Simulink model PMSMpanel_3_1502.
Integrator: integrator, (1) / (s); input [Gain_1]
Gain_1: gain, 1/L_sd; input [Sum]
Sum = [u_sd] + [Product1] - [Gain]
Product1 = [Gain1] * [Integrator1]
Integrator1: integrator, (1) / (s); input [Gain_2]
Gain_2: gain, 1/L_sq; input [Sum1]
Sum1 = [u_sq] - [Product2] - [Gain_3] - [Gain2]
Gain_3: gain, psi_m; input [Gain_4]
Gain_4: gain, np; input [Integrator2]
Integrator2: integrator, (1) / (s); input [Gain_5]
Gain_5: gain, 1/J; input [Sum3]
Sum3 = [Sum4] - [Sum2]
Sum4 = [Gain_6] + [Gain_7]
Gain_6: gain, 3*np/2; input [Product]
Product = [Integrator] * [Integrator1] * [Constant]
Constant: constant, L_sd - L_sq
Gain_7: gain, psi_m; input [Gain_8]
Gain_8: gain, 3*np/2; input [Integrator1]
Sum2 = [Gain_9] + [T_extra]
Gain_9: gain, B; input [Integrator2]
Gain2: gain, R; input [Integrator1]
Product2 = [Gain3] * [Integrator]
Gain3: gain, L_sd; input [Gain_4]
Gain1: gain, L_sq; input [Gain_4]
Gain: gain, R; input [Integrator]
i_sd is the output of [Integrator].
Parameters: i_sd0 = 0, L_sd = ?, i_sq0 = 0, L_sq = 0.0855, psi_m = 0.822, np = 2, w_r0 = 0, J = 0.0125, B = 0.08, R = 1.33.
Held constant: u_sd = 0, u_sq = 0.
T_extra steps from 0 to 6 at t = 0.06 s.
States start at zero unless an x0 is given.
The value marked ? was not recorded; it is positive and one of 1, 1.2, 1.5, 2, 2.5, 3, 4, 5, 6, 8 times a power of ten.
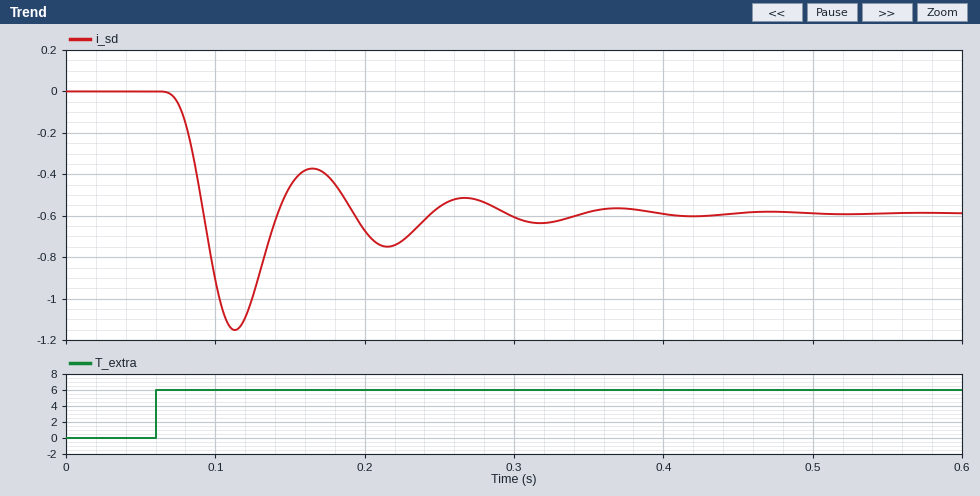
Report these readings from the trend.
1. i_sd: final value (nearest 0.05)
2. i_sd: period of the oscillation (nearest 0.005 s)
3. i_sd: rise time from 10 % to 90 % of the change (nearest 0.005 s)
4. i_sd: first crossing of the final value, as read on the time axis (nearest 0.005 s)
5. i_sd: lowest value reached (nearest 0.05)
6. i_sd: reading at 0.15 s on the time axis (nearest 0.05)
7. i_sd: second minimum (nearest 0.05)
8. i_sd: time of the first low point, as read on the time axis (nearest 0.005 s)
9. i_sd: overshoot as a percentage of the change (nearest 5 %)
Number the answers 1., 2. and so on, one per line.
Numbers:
1. -0.60
2. 0.100 s
3. 0.015 s
4. 0.090 s
5. -1.15
6. -0.45
7. -0.75
8. 0.115 s
9. 95 %
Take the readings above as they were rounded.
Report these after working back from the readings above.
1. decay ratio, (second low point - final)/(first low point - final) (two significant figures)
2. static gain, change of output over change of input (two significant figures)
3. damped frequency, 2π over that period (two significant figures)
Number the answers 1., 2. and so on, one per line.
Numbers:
1. 0.27
2. -0.10
3. 63 rad/s
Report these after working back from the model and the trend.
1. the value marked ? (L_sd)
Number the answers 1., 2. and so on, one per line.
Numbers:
1. 0.06
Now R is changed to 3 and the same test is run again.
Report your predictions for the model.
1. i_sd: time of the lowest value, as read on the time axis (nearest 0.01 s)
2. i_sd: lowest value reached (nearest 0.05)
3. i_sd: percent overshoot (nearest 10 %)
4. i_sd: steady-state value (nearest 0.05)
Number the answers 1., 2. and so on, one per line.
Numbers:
1. 0.12 s
2. -0.85
3. 60 %
4. -0.55
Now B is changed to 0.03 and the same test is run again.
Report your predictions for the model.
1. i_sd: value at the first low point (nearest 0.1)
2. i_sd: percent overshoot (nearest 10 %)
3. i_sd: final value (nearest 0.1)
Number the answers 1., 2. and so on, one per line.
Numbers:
1. -1.3
2. 110 %
3. -0.6
